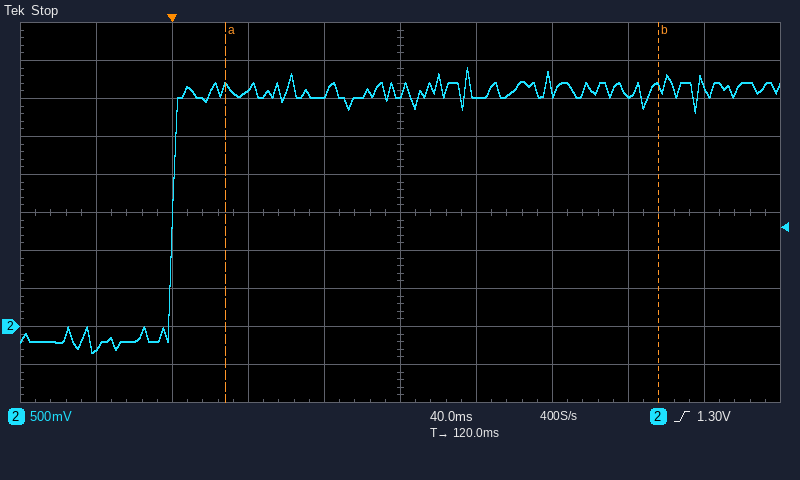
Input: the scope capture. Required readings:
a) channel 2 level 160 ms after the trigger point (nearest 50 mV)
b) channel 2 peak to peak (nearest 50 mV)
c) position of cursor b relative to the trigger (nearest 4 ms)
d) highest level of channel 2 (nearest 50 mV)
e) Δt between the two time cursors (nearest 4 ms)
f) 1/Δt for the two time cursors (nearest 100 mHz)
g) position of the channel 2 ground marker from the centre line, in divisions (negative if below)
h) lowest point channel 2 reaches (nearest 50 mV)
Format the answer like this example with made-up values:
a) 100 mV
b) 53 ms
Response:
a) 3.00 V
b) 3.75 V
c) +256 ms
d) 3.40 V
e) 228 ms
f) 4.4 Hz
g) -3.0 div
h) -350 mV
